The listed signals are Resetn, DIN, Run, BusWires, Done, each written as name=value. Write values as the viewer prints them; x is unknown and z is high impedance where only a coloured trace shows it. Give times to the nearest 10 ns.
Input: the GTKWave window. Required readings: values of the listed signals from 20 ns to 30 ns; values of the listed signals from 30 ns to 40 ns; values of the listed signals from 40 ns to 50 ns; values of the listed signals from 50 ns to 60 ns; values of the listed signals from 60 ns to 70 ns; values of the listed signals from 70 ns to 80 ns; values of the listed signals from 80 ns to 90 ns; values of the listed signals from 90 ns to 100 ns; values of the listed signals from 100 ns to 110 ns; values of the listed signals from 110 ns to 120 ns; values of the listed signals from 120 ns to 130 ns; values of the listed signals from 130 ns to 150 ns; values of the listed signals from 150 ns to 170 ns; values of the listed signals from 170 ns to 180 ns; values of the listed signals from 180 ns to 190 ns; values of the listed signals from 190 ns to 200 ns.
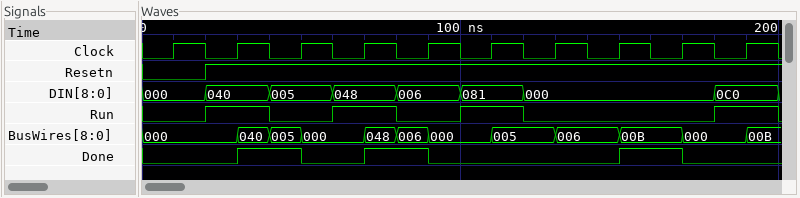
Resetn=1, DIN=040, Run=1, BusWires=000, Done=0
Resetn=1, DIN=040, Run=1, BusWires=040, Done=1
Resetn=1, DIN=005, Run=0, BusWires=005, Done=1
Resetn=1, DIN=005, Run=0, BusWires=000, Done=0
Resetn=1, DIN=048, Run=1, BusWires=000, Done=0
Resetn=1, DIN=048, Run=1, BusWires=048, Done=1
Resetn=1, DIN=006, Run=0, BusWires=006, Done=1
Resetn=1, DIN=006, Run=0, BusWires=000, Done=0
Resetn=1, DIN=081, Run=1, BusWires=000, Done=0
Resetn=1, DIN=081, Run=1, BusWires=005, Done=0
Resetn=1, DIN=000, Run=0, BusWires=005, Done=0
Resetn=1, DIN=000, Run=0, BusWires=006, Done=0
Resetn=1, DIN=000, Run=0, BusWires=00B, Done=1
Resetn=1, DIN=000, Run=0, BusWires=000, Done=0
Resetn=1, DIN=0C0, Run=1, BusWires=000, Done=0
Resetn=1, DIN=0C0, Run=1, BusWires=00B, Done=0
